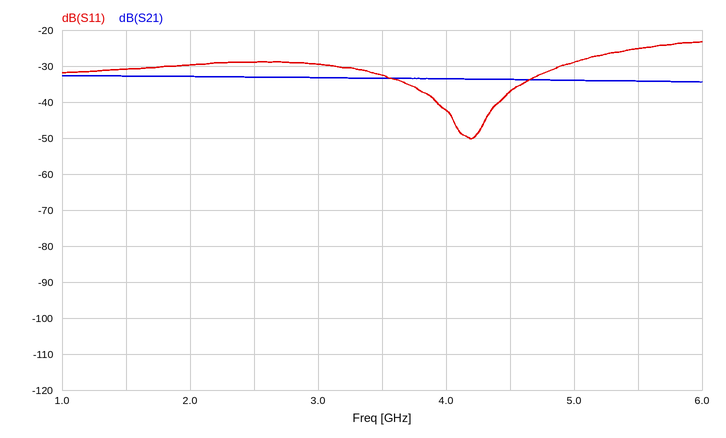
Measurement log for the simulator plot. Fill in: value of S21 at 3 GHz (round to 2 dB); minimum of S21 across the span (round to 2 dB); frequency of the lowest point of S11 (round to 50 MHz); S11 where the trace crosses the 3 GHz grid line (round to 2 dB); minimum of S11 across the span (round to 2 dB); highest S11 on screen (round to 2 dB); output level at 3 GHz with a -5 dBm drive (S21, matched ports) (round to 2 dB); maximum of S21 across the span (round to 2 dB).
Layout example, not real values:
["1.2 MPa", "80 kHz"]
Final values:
["-34 dB", "-34 dB", "4.20 GHz", "-30 dB", "-50 dB", "-24 dB", "-38 dBm", "-32 dB"]
